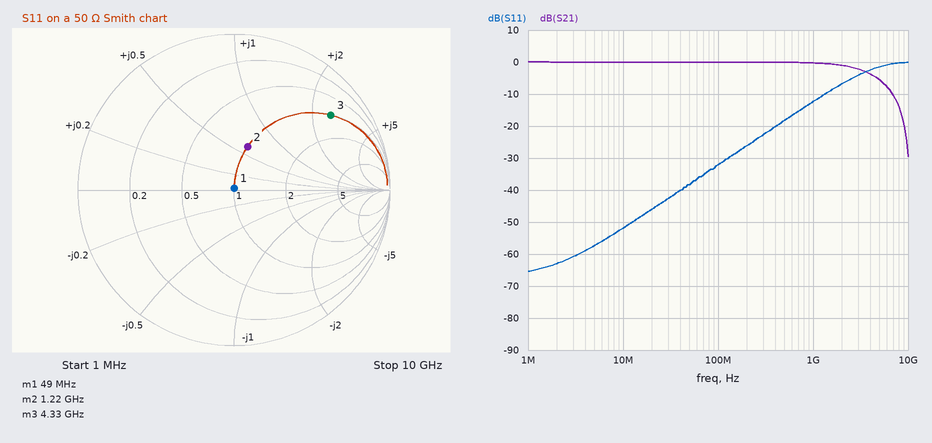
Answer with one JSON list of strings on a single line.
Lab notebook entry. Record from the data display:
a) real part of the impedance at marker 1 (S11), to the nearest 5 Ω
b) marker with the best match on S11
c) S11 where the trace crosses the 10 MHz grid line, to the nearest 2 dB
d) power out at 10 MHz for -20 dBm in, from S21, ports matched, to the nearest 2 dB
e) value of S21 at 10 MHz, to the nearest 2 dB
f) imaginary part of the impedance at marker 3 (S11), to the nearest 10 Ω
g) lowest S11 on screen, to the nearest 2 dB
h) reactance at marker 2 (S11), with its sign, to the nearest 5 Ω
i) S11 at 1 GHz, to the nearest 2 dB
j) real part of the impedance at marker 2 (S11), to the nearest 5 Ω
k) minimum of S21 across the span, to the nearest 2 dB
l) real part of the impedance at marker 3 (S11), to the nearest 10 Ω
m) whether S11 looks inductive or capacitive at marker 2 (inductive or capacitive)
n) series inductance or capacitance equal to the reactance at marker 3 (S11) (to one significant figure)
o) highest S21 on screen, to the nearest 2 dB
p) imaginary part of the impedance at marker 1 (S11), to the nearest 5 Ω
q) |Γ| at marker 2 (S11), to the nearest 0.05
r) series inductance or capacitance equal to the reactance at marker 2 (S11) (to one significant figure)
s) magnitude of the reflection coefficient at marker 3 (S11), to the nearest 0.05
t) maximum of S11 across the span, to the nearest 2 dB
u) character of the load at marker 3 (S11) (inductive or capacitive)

["50 Ω", "marker 1", "-52 dB", "-20 dBm", "0 dB", "+130 Ω", "-66 dB", "+30 Ω", "-12 dB", "50 Ω", "-30 dB", "50 Ω", "inductive", "5 nH", "0 dB", "0 Ω", "0.30", "4 nH", "0.80", "0 dB", "inductive"]
